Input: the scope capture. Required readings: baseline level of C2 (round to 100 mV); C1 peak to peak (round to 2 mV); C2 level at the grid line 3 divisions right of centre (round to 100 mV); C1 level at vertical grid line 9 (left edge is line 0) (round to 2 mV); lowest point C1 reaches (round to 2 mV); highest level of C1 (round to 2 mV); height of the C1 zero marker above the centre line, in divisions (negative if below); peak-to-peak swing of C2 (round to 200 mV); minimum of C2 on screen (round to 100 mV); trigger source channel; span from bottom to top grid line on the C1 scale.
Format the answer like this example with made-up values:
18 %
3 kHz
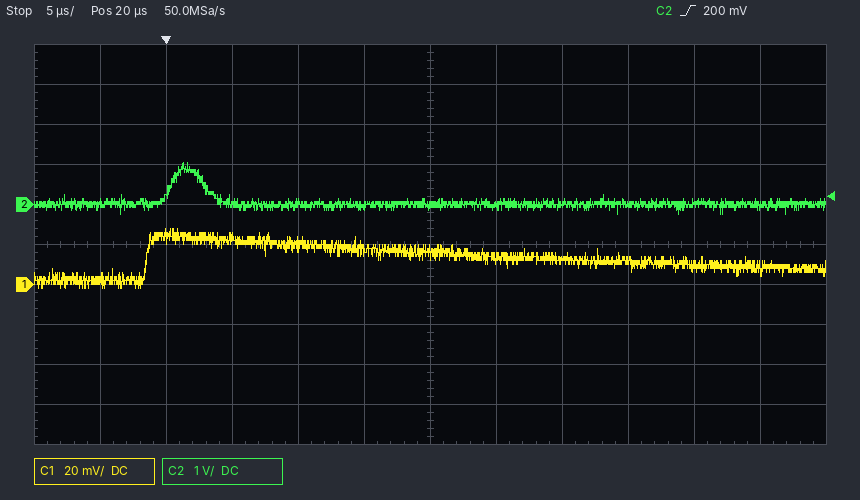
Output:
0.0 V
30 mV
0.0 V
12 mV
-2 mV
28 mV
-1.0 div
1.2 V
-200 mV
C2
200 mV
